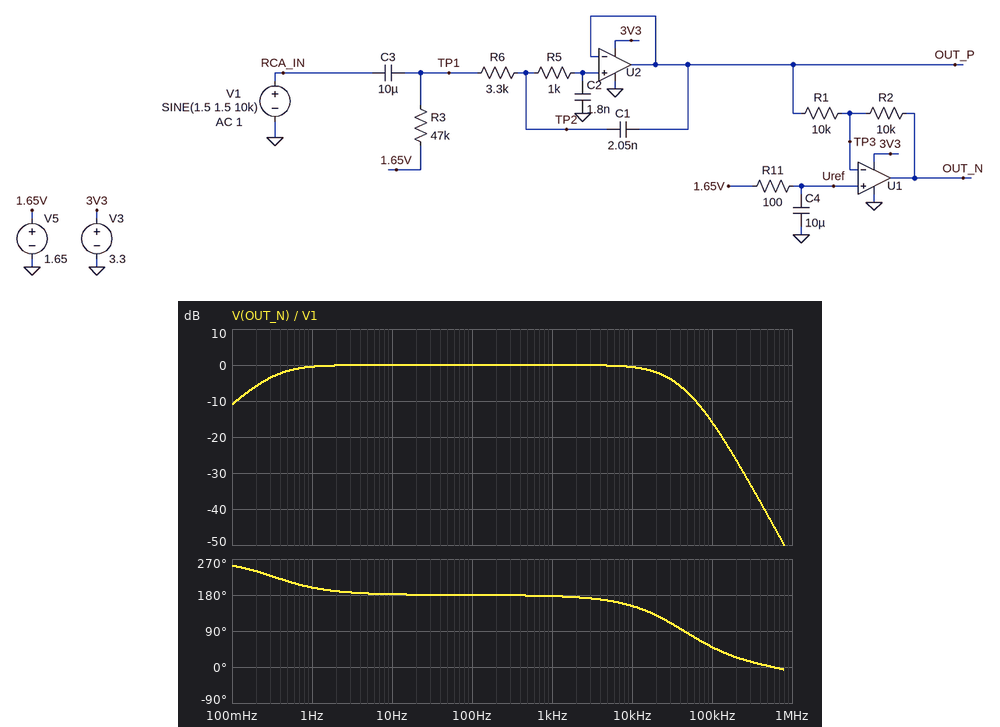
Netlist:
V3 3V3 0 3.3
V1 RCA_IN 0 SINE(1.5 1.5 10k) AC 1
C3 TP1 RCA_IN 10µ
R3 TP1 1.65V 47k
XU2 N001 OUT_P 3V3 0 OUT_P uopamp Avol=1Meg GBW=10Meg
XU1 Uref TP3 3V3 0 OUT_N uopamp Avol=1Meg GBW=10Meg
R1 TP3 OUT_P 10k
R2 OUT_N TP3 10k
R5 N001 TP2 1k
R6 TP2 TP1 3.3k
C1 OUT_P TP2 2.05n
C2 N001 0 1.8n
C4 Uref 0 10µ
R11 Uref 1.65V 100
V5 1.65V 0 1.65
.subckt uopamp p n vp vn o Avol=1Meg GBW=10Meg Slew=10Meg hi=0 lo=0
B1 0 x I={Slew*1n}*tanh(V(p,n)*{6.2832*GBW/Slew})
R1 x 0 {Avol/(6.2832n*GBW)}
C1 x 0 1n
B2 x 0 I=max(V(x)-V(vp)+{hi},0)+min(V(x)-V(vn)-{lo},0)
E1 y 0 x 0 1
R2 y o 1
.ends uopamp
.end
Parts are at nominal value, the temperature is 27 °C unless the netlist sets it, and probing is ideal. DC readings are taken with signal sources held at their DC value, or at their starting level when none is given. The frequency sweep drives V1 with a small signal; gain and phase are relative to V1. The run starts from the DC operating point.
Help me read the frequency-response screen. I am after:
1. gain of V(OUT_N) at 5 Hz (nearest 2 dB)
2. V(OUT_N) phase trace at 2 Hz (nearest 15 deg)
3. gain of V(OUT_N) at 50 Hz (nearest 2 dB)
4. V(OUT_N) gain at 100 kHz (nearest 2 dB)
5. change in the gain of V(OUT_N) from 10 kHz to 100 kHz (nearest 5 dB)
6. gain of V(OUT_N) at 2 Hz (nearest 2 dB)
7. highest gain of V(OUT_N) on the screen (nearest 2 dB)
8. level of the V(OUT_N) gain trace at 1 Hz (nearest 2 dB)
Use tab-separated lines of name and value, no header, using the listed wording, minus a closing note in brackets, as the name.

gain of V(OUT_N) at 5 Hz	0 dB
V(OUT_N) phase trace at 2 Hz	195 deg
gain of V(OUT_N) at 50 Hz	0 dB
V(OUT_N) gain at 100 kHz	-16 dB
change in the gain of V(OUT_N) from 10 kHz to 100 kHz	-15 dB
gain of V(OUT_N) at 2 Hz	0 dB
highest gain of V(OUT_N) on the screen	0 dB
level of the V(OUT_N) gain trace at 1 Hz	0 dB
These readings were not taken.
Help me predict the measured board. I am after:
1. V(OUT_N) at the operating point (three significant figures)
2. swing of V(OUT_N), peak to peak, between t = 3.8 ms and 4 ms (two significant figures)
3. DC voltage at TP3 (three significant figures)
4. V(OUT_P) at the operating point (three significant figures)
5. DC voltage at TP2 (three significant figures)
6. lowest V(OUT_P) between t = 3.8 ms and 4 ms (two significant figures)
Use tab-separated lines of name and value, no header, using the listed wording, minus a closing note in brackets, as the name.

V(OUT_N) at the operating point	1.65 V
swing of V(OUT_N), peak to peak, between t = 3.8 ms and 4 ms	2.8 V
DC voltage at TP3	1.65 V
V(OUT_P) at the operating point	1.65 V
DC voltage at TP2	1.65 V
lowest V(OUT_P) between t = 3.8 ms and 4 ms	250 mV
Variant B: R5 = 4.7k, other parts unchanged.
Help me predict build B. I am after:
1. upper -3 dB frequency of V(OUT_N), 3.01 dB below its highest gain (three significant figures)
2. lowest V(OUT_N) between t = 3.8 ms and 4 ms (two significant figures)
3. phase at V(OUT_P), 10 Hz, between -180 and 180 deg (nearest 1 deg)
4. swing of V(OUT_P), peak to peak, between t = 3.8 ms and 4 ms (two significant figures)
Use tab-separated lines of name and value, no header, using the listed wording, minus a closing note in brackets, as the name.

upper -3 dB frequency of V(OUT_N), 3.01 dB below its highest gain	14.5 kHz
lowest V(OUT_N) between t = 3.8 ms and 4 ms	390 mV
phase at V(OUT_P), 10 Hz, between -180 and 180 deg	2 deg
swing of V(OUT_P), peak to peak, between t = 3.8 ms and 4 ms	2.5 V
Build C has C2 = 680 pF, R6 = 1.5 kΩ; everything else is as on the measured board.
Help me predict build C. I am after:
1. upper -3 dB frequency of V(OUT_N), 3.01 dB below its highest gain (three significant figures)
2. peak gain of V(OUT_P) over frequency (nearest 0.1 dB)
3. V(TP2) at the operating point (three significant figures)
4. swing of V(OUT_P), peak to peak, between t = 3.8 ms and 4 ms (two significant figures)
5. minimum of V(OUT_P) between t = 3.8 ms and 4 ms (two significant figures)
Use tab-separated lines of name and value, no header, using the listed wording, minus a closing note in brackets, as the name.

upper -3 dB frequency of V(OUT_N), 3.01 dB below its highest gain	123 kHz
peak gain of V(OUT_P) over frequency	0.5 dB
V(TP2) at the operating point	1.65 V
swing of V(OUT_P), peak to peak, between t = 3.8 ms and 4 ms	3.0 V
minimum of V(OUT_P) between t = 3.8 ms and 4 ms	150 mV
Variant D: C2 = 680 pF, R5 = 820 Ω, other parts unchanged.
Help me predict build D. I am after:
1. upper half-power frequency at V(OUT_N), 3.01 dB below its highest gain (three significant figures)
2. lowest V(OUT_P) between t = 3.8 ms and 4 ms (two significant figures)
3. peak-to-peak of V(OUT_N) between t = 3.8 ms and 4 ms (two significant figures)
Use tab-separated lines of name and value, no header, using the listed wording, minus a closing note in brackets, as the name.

upper half-power frequency at V(OUT_N), 3.01 dB below its highest gain	80.3 kHz
lowest V(OUT_P) between t = 3.8 ms and 4 ms	150 mV
peak-to-peak of V(OUT_N) between t = 3.8 ms and 4 ms	3.0 V
